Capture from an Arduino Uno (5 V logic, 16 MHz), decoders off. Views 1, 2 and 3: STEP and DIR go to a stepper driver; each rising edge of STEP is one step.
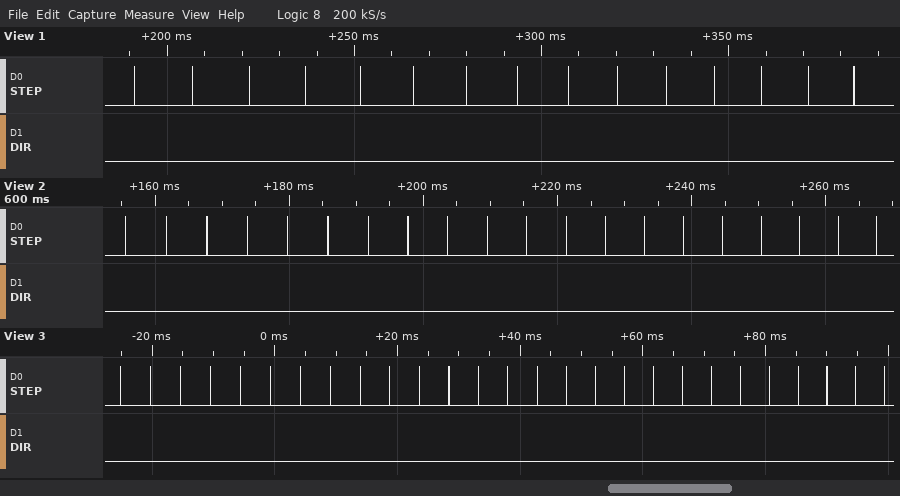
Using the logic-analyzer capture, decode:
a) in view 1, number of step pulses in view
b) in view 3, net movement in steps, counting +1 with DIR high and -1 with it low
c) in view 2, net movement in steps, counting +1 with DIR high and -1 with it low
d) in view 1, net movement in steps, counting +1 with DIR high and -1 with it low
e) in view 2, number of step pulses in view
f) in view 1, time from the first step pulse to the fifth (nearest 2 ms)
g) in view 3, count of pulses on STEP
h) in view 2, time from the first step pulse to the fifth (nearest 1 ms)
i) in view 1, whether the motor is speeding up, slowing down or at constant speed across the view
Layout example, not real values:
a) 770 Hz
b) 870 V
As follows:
a) 15
b) -27
c) -20
d) -15
e) 20
f) 60 ms
g) 27
h) 24 ms
i) speeding up
